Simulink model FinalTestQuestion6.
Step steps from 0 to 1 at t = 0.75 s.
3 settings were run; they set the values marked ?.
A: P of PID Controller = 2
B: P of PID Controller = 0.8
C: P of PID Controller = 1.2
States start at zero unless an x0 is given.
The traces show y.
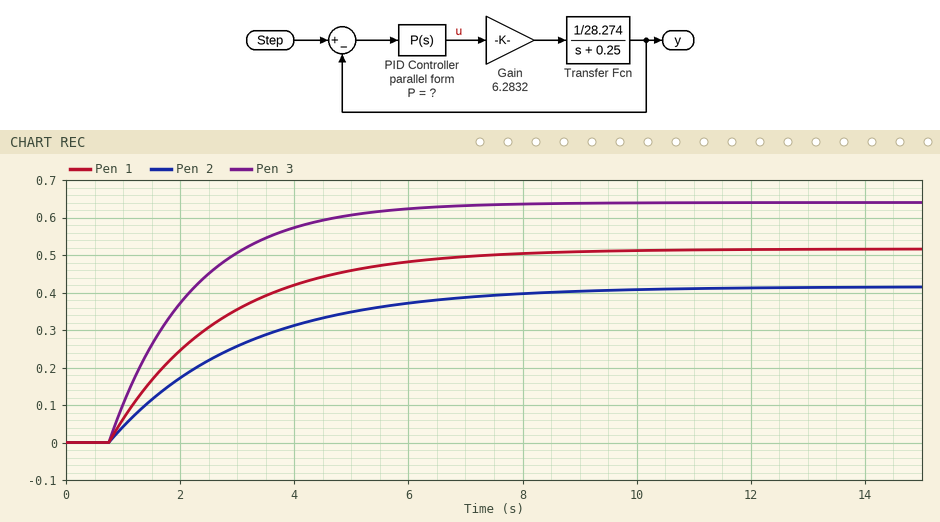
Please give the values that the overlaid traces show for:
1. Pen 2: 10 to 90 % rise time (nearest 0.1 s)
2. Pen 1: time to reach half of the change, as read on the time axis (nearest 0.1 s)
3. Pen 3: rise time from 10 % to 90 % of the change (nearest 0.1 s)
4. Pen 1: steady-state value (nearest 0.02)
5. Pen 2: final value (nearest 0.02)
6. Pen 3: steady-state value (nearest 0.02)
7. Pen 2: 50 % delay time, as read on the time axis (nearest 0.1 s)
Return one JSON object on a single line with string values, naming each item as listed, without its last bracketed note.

{"Pen 2: 10 to 90 % rise time": "5.1 s", "Pen 1: time to reach half of the change, as read on the time axis": "2.1 s", "Pen 3: rise time from 10 % to 90 % of the change": "3.2 s", "Pen 1: steady-state value": "0.52", "Pen 2: final value": "0.42", "Pen 3: steady-state value": "0.64", "Pen 2: 50 % delay time, as read on the time axis": "2.4 s"}
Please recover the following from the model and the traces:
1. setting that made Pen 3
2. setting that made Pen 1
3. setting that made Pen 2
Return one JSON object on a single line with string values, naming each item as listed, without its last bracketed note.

{"setting that made Pen 3": "A", "setting that made Pen 1": "C", "setting that made Pen 2": "B"}
